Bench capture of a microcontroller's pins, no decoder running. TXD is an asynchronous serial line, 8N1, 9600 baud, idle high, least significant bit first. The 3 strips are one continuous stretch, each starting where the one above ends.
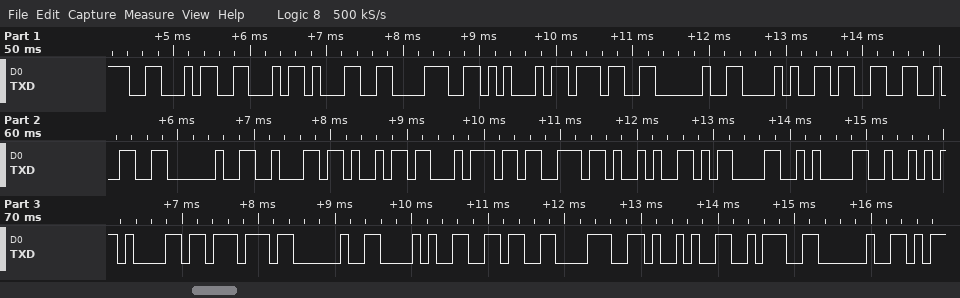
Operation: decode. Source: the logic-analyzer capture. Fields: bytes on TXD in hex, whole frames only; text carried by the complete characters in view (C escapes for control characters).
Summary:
46 46 31 38 45 37 20 28 33 32 20 62 69 74 73 29 0D 0A 52 61 77 20 28 36 38 29 3A 20
"FF18E7 (32 bits)\r\nRaw (68): "
